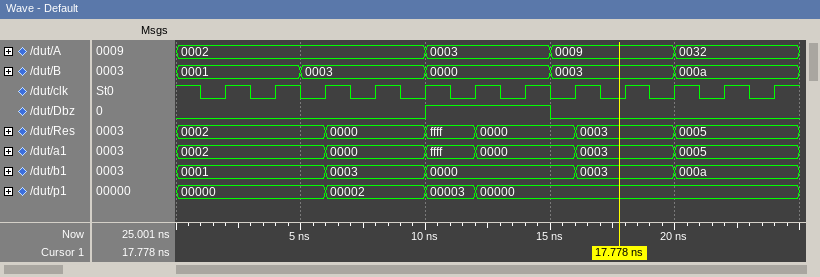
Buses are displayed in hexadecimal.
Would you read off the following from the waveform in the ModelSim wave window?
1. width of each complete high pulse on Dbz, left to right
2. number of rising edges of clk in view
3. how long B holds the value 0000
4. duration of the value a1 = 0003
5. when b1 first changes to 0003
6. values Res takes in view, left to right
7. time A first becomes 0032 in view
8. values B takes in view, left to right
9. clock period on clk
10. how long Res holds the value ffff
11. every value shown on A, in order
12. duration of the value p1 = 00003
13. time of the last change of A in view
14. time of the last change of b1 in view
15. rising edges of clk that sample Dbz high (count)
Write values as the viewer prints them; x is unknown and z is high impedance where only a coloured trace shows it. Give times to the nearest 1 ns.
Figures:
5 ns
12
5 ns
4 ns
6 ns
0002, 0000, ffff, 0000, 0003, 0005
20 ns
0001, 0003, 0000, 0003, 000a
2 ns
2 ns
0002, 0003, 0009, 0032
2 ns
20 ns
20 ns
2
